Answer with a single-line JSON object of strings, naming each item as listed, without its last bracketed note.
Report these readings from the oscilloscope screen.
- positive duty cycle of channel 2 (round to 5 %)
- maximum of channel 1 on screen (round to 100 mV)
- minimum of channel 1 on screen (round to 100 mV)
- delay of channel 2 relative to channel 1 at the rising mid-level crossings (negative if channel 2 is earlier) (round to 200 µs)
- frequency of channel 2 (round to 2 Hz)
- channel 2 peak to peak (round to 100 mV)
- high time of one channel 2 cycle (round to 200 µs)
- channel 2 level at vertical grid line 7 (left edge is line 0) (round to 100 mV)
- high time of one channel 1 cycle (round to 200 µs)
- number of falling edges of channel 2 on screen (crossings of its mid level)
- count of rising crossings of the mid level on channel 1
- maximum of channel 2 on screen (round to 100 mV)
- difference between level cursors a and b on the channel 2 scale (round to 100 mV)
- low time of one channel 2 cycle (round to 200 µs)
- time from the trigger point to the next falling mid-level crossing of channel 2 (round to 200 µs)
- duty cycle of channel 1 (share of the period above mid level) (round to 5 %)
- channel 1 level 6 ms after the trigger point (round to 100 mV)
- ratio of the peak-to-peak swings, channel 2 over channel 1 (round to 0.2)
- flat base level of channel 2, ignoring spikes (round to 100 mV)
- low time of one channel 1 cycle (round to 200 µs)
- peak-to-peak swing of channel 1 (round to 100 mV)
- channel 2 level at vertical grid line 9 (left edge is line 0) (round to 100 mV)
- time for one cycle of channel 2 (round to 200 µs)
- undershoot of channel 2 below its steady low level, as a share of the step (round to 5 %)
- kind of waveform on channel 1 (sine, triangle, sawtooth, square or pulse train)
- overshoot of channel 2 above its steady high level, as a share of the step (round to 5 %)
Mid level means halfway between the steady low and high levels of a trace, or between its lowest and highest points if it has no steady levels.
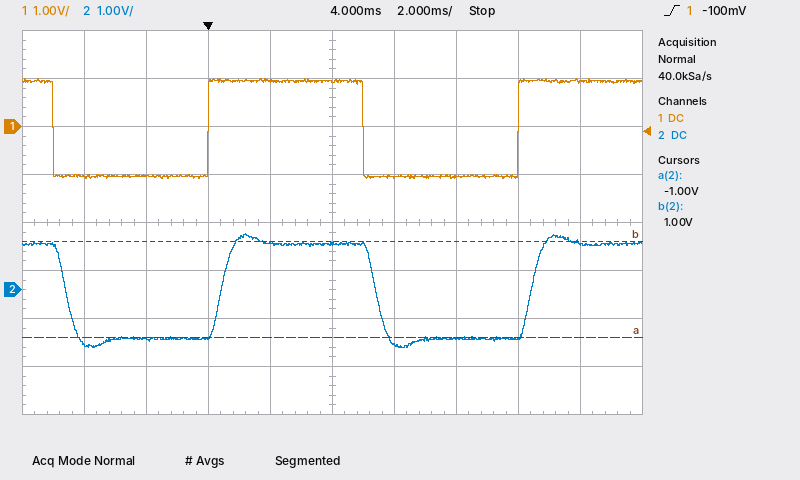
{"positive duty cycle of channel 2": "50 %", "maximum of channel 1 on screen": "1.0 V", "minimum of channel 1 on screen": "-1.1 V", "delay of channel 2 relative to channel 1 at the rising mid-level crossings (negative if channel 2 is earlier)": "+400 µs", "frequency of channel 2": "100 Hz", "channel 2 peak to peak": "2.4 V", "high time of one channel 2 cycle": "5.0 ms", "channel 2 level at vertical grid line 7 (left edge is line 0)": "-1.0 V", "high time of one channel 1 cycle": "5.0 ms", "number of falling edges of channel 2 on screen": "2", "count of rising crossings of the mid level on channel 1": "2", "maximum of channel 2 on screen": "1.2 V", "difference between level cursors a and b on the channel 2 scale": "2.0 V", "low time of one channel 2 cycle": "5.0 ms", "time from the trigger point to the next falling mid-level crossing of channel 2": "5.4 ms", "duty cycle of channel 1 (share of the period above mid level)": "50 %", "channel 1 level 6 ms after the trigger point": "-1.1 V", "ratio of the peak-to-peak swings, channel 2 over channel 1": "1.2", "flat base level of channel 2, ignoring spikes": "-1.0 V", "low time of one channel 1 cycle": "5.0 ms", "peak-to-peak swing of channel 1": "2.1 V", "channel 2 level at vertical grid line 9 (left edge is line 0)": "1.0 V", "time for one cycle of channel 2": "10.0 ms", "undershoot of channel 2 below its steady low level, as a share of the step": "10 %", "kind of waveform on channel 1": "square", "overshoot of channel 2 above its steady high level, as a share of the step": "10 %"}
